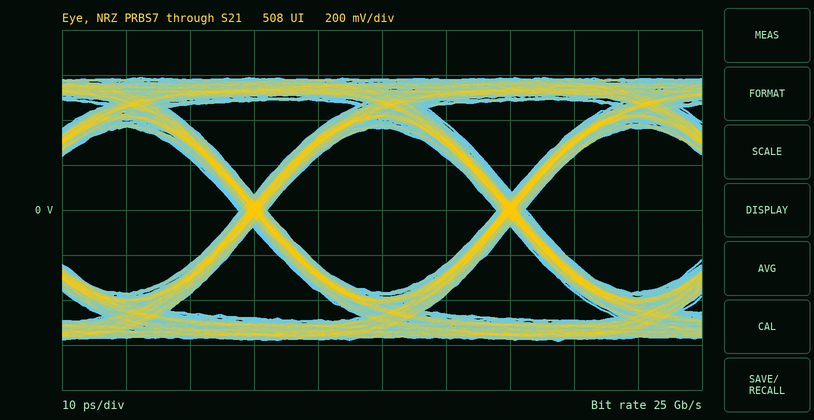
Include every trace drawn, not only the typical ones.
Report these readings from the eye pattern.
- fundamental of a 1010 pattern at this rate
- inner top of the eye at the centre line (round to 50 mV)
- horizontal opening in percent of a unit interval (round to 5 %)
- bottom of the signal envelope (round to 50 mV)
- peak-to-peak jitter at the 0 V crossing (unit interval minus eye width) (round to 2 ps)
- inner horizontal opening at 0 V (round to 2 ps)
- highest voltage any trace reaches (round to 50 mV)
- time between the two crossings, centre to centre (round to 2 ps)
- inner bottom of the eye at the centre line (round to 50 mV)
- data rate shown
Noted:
12.5 GHz
350 mV
90 %
-600 mV
4 ps
36 ps
600 mV
40 ps
-350 mV
25 Gb/s
